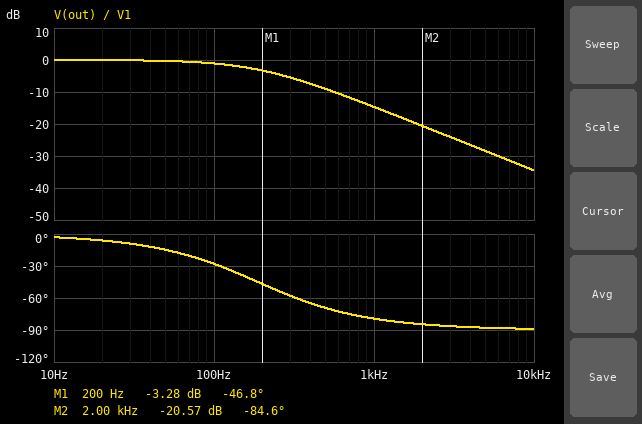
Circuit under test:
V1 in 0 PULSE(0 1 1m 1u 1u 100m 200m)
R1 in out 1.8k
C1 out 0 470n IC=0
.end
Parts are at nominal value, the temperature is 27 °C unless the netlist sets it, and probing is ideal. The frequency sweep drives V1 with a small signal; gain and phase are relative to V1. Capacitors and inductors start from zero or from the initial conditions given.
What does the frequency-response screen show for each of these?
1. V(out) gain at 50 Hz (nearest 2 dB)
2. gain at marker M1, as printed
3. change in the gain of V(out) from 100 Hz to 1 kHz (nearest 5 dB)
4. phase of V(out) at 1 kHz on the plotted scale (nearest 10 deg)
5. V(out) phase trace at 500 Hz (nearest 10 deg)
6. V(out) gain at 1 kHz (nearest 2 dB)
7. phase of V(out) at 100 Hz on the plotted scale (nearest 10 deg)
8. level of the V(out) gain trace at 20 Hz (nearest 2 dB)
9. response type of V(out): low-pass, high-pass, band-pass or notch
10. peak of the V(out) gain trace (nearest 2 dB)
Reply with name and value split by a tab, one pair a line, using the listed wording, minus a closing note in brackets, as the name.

V(out) gain at 50 Hz	0 dB
gain at marker M1, as printed	-3.28 dB
change in the gain of V(out) from 100 Hz to 1 kHz	-15 dB
phase of V(out) at 1 kHz on the plotted scale	-80 deg
V(out) phase trace at 500 Hz	-70 deg
V(out) gain at 1 kHz	-14 dB
phase of V(out) at 100 Hz on the plotted scale	-30 deg
level of the V(out) gain trace at 20 Hz	0 dB
response type of V(out): low-pass, high-pass, band-pass or notch	low-pass
peak of the V(out) gain trace	0 dB
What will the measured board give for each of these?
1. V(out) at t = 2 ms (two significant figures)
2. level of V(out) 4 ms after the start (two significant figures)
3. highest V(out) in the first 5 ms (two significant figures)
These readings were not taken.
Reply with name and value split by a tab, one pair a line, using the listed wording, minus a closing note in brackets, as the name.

V(out) at t = 2 ms	690 mV
level of V(out) 4 ms after the start	970 mV
highest V(out) in the first 5 ms	990 mV
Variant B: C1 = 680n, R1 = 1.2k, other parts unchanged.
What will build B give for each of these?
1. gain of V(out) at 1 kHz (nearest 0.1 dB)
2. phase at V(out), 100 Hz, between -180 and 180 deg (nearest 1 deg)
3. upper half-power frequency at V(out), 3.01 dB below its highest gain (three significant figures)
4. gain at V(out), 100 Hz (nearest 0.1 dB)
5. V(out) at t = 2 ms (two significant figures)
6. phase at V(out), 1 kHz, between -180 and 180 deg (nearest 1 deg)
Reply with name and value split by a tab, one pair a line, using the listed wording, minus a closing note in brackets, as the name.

gain of V(out) at 1 kHz	-14.4 dB
phase at V(out), 100 Hz, between -180 and 180 deg	-27 deg
upper half-power frequency at V(out), 3.01 dB below its highest gain	195 Hz
gain at V(out), 100 Hz	-1.0 dB
V(out) at t = 2 ms	710 mV
phase at V(out), 1 kHz, between -180 and 180 deg	-79 deg
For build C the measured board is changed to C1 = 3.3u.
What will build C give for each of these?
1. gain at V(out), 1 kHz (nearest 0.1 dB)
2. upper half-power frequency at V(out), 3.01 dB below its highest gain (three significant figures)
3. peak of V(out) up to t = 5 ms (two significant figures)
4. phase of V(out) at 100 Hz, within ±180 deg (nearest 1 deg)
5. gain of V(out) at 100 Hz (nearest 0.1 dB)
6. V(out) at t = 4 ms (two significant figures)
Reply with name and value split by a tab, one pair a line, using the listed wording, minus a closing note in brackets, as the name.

gain at V(out), 1 kHz	-31.4 dB
upper half-power frequency at V(out), 3.01 dB below its highest gain	26.8 Hz
peak of V(out) up to t = 5 ms	490 mV
phase of V(out) at 100 Hz, within ±180 deg	-75 deg
gain of V(out) at 100 Hz	-11.7 dB
V(out) at t = 4 ms	400 mV
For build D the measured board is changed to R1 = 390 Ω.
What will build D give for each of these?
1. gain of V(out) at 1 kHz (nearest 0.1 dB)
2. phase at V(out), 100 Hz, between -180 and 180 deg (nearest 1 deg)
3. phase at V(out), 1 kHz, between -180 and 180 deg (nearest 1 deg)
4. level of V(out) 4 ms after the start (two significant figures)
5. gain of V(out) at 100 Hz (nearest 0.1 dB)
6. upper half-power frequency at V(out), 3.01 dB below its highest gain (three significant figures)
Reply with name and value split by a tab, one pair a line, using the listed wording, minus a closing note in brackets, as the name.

gain of V(out) at 1 kHz	-3.7 dB
phase at V(out), 100 Hz, between -180 and 180 deg	-7 deg
phase at V(out), 1 kHz, between -180 and 180 deg	-49 deg
level of V(out) 4 ms after the start	1.0 V
gain of V(out) at 100 Hz	-0.1 dB
upper half-power frequency at V(out), 3.01 dB below its highest gain	868 Hz
